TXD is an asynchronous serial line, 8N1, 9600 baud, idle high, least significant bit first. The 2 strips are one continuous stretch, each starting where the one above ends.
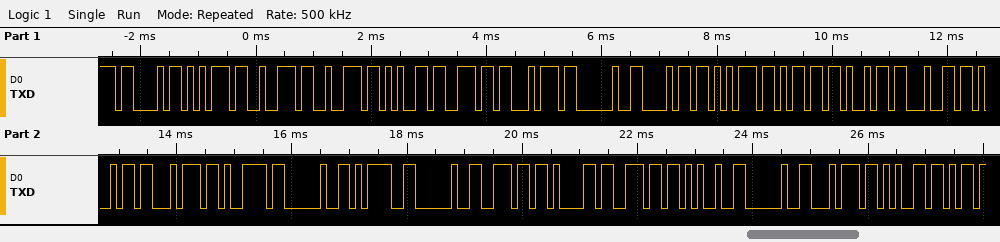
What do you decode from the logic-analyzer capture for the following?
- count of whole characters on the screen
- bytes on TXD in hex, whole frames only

26
0x43 0x75 0x72 0x72 0x65 0x6E 0x74 0x20 0x68 0x75 0x6D 0x69 0x64 0x69 0x74 0x79 0x20 0x3D 0x20 0x6E 0x61 0x6E 0x25 0x20 0x74 0x65
